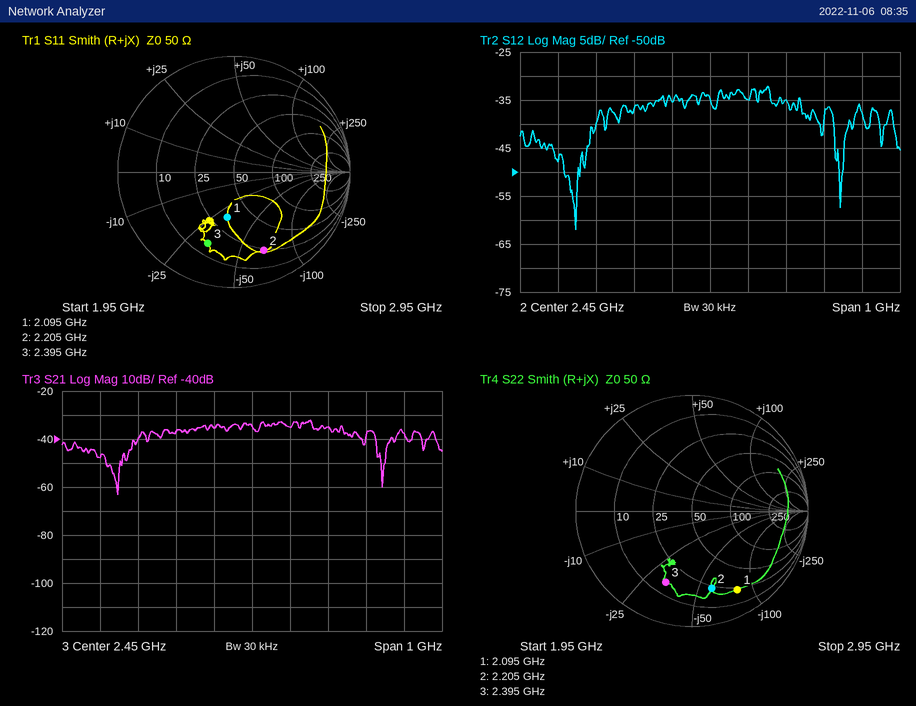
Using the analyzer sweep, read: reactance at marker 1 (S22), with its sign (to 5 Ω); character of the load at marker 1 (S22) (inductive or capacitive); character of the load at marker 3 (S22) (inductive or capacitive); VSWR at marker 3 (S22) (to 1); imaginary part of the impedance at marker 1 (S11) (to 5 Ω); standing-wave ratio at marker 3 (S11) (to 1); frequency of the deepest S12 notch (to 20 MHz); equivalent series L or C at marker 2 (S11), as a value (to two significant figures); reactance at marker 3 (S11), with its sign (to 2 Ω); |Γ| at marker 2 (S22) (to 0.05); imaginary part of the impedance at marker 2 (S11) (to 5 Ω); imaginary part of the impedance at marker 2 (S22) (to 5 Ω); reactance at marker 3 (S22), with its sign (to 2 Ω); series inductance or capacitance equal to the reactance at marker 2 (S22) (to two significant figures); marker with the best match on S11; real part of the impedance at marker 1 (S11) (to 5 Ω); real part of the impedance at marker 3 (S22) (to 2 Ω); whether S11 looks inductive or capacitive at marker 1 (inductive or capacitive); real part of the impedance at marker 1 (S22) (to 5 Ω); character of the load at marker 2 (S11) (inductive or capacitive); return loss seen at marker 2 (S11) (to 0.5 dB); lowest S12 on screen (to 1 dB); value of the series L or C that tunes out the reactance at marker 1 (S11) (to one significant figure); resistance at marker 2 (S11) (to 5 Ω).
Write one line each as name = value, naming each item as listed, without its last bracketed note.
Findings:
reactance at marker 1 (S22), with its sign = -80 Ω
character of the load at marker 1 (S22) = capacitive
character of the load at marker 3 (S22) = capacitive
VSWR at marker 3 (S22) = 5
imaginary part of the impedance at marker 1 (S11) = -30 Ω
standing-wave ratio at marker 3 (S11) = 5
frequency of the deepest S12 notch = 2.10 GHz
equivalent series L or C at marker 2 (S11), as a value = 1.1 pF
reactance at marker 3 (S11), with its sign = -32 Ω
|Γ| at marker 2 (S22) = 0.70
imaginary part of the impedance at marker 2 (S11) = -65 Ω
imaginary part of the impedance at marker 2 (S22) = -60 Ω
reactance at marker 3 (S22), with its sign = -32 Ω
series inductance or capacitance equal to the reactance at marker 2 (S22) = 1.2 pF
marker with the best match on S11 = marker 1
real part of the impedance at marker 1 (S11) = 35 Ω
real part of the impedance at marker 3 (S22) = 16 Ω
whether S11 looks inductive or capacitive at marker 1 = capacitive
real part of the impedance at marker 1 (S22) = 25 Ω
character of the load at marker 2 (S11) = capacitive
return loss seen at marker 2 (S11) = 3.0 dB
lowest S12 on screen = -62 dB
value of the series L or C that tunes out the reactance at marker 1 (S11) = 2 nH
resistance at marker 2 (S11) = 25 Ω
